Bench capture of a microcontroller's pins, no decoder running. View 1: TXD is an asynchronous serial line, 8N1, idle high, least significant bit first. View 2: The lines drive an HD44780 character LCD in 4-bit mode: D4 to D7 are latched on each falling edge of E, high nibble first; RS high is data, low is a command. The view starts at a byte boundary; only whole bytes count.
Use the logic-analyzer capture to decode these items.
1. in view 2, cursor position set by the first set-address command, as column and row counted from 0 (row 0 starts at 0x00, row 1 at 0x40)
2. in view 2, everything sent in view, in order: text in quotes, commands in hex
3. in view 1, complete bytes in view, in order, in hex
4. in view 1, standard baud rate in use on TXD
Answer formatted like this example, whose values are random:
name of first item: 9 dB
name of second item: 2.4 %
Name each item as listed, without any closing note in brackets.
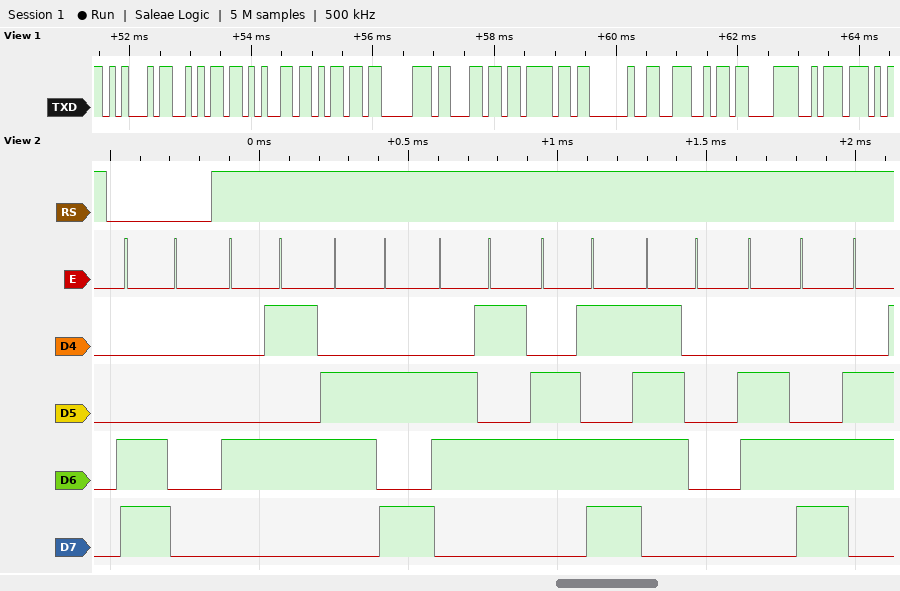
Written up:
in view 2, cursor position set by the first set-address command, as column and row counted from 0: column 0, row 1
in view 2, everything sent in view, in order: text in quotes, commands in hex: 0xC0 "Ejempl"
in view 1, complete bytes in view, in order, in hex: 0x45 0x6A 0x65 0x6D 0x70 0x6C 0x6F 0x20 0x4E 0xC3 0xBA
in view 1, standard baud rate in use on TXD: 9600 baud
